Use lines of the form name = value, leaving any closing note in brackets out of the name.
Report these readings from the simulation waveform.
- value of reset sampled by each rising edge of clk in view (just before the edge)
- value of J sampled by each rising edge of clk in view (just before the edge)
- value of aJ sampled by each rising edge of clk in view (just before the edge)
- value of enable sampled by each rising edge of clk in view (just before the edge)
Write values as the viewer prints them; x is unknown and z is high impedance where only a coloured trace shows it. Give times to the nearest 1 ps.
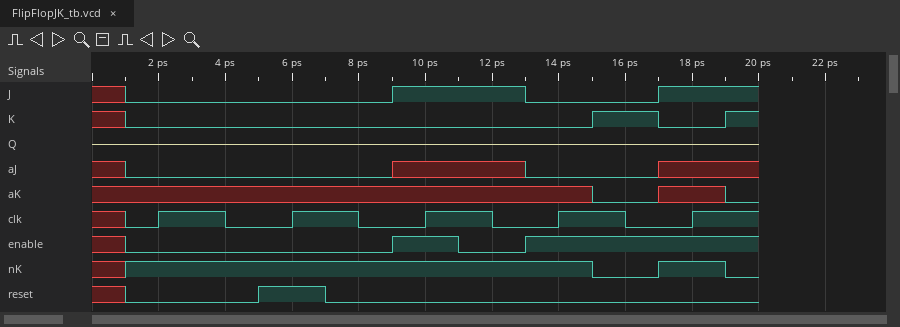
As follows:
value of reset sampled by each rising edge of clk in view = 0 1 0 0 0
value of J sampled by each rising edge of clk in view = 0 0 1 0 1
value of aJ sampled by each rising edge of clk in view = 0 0 x 0 x
value of enable sampled by each rising edge of clk in view = 0 0 1 1 1
